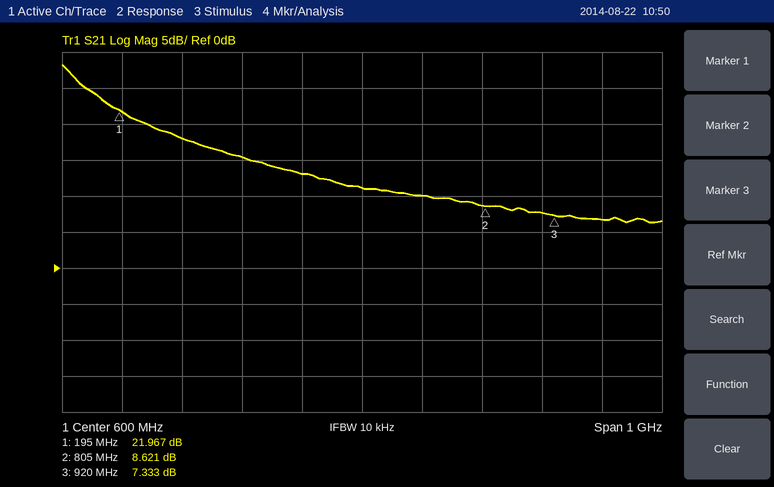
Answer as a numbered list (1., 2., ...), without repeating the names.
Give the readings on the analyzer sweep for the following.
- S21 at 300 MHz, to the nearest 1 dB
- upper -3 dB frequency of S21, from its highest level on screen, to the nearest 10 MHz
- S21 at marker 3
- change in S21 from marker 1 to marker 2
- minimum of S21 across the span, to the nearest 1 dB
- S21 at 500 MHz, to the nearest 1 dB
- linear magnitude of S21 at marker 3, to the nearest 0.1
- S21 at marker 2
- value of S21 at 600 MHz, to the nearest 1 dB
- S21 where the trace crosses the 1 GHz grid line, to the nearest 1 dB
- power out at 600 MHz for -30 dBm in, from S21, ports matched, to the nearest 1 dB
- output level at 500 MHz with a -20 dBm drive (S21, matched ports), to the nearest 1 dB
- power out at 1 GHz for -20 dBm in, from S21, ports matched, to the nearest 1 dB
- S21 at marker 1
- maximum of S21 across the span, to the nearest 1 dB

1. 18 dB
2. 140 MHz
3. 7.333 dB
4. -13.346 dB
5. 6 dB
6. 13 dB
7. 2.3
8. 8.621 dB
9. 11 dB
10. 7 dB
11. -19 dBm
12. -7 dBm
13. -13 dBm
14. 21.967 dB
15. 28 dB
